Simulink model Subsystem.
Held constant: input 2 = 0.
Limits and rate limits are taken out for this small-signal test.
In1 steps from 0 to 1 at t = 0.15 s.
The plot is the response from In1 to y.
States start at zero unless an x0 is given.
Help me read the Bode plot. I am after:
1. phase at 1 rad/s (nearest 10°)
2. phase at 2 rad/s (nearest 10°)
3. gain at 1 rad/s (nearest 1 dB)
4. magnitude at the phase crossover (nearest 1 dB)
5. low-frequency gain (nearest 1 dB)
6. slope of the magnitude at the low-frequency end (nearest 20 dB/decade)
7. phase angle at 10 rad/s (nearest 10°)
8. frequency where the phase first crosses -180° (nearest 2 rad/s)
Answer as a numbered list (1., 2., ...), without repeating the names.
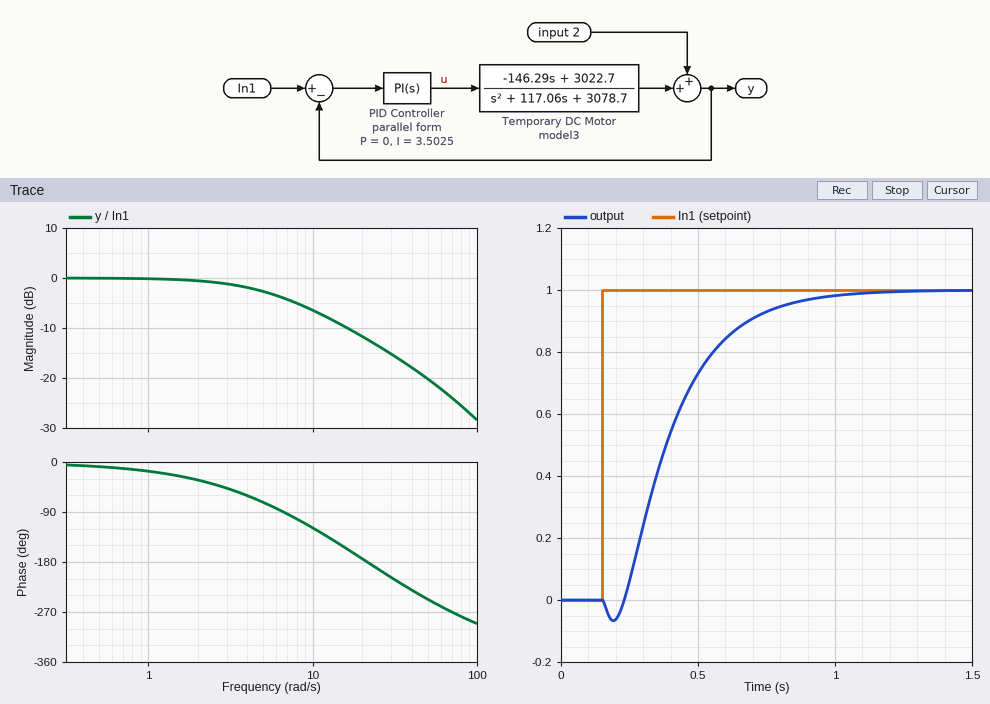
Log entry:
1. -20°
2. -30°
3. 0 dB
4. -12 dB
5. 0 dB
6. 0 dB/decade
7. -120°
8. 22 rad/s
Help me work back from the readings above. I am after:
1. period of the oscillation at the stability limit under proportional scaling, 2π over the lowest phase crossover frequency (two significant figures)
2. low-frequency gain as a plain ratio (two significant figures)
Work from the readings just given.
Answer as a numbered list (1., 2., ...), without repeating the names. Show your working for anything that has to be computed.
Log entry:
1. 2π / 22 = 0.29 s
2. 10^(0 / 20) = 1.0
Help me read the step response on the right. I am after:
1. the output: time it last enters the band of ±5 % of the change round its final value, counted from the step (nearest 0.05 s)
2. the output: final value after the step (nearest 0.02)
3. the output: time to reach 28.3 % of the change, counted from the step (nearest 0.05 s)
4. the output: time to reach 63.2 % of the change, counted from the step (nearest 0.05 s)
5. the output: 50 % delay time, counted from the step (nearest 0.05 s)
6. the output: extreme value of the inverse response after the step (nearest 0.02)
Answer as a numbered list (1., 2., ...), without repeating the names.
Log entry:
1. 0.65 s
2. 1.00
3. 0.15 s
4. 0.30 s
5. 0.25 s
6. -0.06
